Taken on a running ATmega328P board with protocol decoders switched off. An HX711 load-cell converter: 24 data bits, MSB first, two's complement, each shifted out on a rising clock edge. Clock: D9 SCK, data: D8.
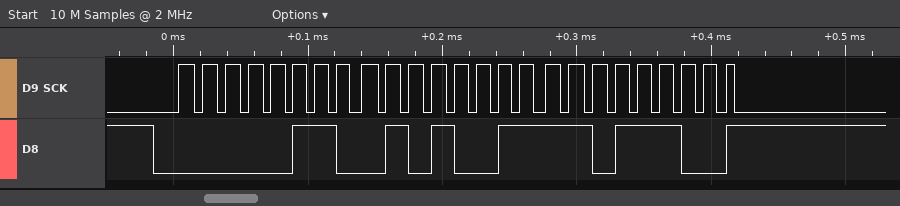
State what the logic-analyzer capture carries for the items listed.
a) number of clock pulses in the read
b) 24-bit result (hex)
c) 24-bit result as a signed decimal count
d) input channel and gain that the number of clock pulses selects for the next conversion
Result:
25
0x0653DC
414684
channel A, gain 128
